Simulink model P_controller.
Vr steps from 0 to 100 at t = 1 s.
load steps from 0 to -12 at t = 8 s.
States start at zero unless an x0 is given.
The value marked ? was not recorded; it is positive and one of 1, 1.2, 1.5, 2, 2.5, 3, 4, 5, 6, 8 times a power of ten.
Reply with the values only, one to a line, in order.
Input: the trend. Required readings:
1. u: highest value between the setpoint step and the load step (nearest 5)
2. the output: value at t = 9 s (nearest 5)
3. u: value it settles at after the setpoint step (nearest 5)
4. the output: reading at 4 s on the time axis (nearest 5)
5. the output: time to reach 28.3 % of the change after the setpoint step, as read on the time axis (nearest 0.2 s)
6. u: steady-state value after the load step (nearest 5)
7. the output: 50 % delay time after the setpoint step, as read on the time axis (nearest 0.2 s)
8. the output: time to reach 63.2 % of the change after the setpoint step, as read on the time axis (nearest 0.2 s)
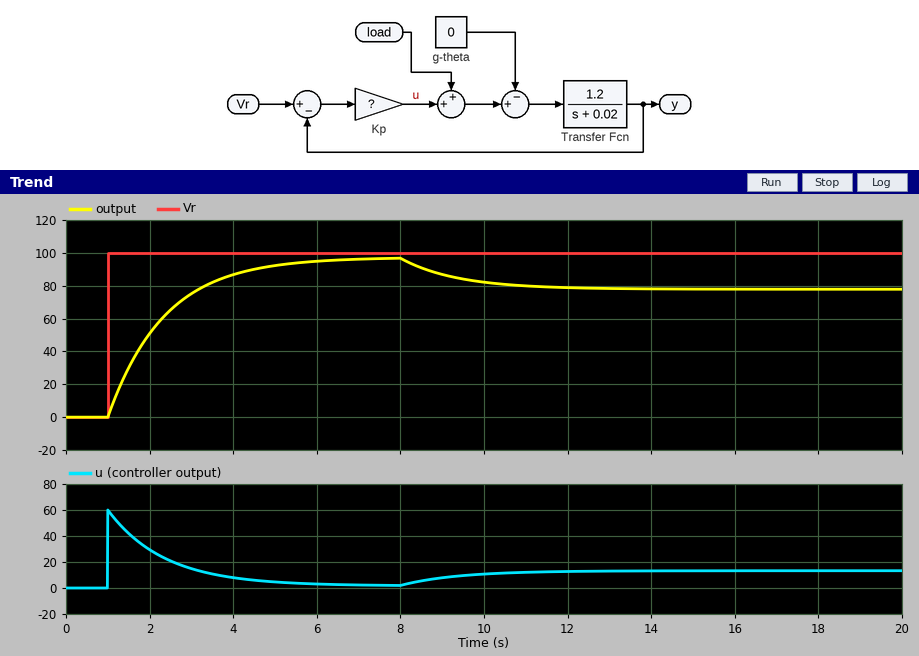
60
85
0
85
1.4 s
15
2.0 s
2.4 s
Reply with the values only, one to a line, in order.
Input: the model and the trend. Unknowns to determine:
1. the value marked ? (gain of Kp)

0.6
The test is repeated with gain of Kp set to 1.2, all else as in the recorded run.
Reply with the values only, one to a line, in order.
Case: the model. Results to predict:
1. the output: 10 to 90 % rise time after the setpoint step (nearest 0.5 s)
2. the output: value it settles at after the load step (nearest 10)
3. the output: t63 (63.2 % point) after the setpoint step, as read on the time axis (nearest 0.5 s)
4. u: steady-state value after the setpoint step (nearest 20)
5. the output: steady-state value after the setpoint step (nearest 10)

1.5 s
90
1.5 s
0
100
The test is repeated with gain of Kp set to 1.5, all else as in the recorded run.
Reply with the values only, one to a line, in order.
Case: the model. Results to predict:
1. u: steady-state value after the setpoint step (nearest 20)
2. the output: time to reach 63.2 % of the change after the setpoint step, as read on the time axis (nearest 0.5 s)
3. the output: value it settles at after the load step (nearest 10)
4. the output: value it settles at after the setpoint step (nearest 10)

0
1.5 s
90
100
